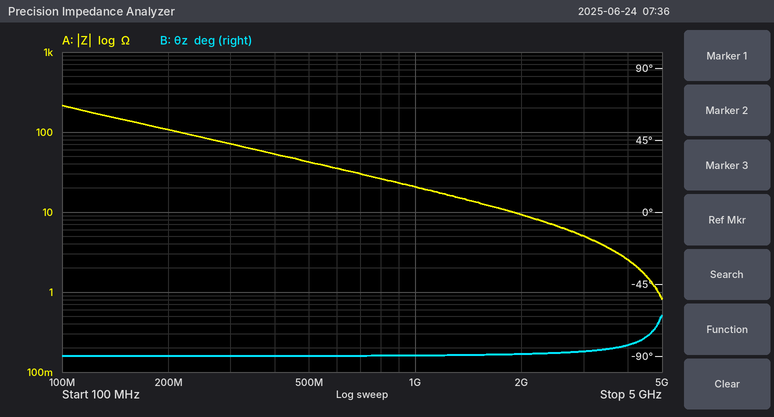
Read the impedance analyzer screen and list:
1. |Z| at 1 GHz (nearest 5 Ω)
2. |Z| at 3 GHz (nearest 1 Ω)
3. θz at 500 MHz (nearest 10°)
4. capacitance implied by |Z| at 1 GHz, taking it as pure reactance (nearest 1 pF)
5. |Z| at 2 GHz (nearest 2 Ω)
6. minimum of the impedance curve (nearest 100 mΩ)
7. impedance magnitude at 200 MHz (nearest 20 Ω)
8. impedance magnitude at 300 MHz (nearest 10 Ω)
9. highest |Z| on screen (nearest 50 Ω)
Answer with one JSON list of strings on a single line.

["20 Ω", "5 Ω", "-90°", "8 pF", "10 Ω", "800 mΩ", "100 Ω", "70 Ω", "200 Ω"]
